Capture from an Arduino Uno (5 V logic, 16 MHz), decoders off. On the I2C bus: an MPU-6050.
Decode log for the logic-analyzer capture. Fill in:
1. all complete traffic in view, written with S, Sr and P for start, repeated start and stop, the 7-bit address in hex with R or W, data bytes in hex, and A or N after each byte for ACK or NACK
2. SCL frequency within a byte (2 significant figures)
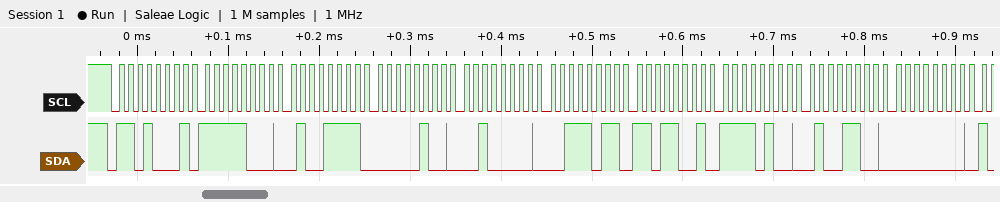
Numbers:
S 68R A F8 A 4F A 04 A 20 A 3B A D9 A F4 A 4C A 00 A
100 kHz
